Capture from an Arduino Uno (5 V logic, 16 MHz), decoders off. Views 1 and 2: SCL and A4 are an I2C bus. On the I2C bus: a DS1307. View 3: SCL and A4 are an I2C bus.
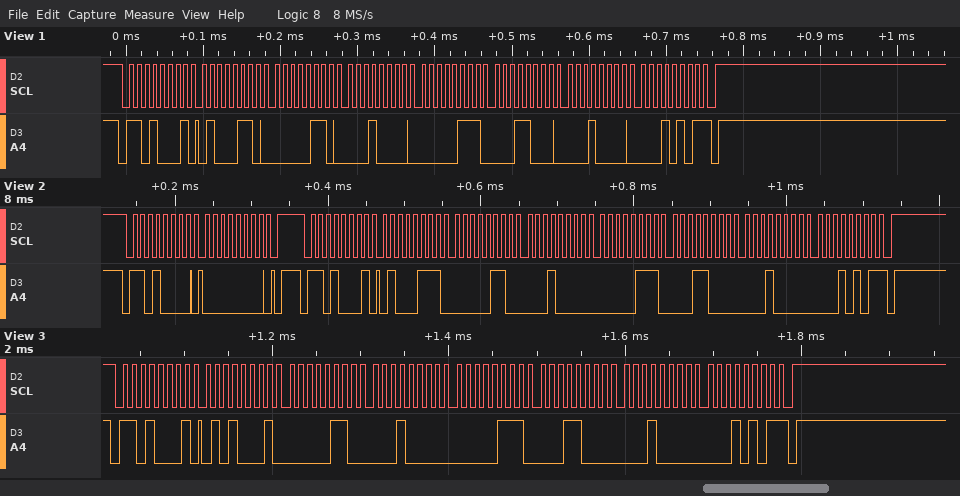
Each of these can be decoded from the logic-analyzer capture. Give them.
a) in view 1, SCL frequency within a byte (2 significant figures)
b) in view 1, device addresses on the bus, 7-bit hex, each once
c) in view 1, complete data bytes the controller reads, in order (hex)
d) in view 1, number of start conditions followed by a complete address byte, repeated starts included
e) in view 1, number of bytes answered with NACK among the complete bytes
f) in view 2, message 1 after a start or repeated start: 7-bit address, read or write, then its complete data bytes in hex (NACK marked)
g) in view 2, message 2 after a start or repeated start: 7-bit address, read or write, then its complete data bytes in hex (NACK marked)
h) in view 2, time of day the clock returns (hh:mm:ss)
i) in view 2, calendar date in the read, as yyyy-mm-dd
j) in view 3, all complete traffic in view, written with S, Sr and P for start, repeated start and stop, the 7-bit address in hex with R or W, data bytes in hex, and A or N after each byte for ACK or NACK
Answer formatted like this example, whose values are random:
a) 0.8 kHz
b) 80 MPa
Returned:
a) 100 kHz
b) 0x68
c) 46 06 10 07 18 10 15
d) 1
e) 1
f) 0x68 write: 00
g) 0x68 read: 47 06 10 07 18 10 15 NACK
h) 10:06:47
i) 2015-10-18
j) S 68R A 51 A 06 A 10 A 07 A 18 A 10 A 15 N P
